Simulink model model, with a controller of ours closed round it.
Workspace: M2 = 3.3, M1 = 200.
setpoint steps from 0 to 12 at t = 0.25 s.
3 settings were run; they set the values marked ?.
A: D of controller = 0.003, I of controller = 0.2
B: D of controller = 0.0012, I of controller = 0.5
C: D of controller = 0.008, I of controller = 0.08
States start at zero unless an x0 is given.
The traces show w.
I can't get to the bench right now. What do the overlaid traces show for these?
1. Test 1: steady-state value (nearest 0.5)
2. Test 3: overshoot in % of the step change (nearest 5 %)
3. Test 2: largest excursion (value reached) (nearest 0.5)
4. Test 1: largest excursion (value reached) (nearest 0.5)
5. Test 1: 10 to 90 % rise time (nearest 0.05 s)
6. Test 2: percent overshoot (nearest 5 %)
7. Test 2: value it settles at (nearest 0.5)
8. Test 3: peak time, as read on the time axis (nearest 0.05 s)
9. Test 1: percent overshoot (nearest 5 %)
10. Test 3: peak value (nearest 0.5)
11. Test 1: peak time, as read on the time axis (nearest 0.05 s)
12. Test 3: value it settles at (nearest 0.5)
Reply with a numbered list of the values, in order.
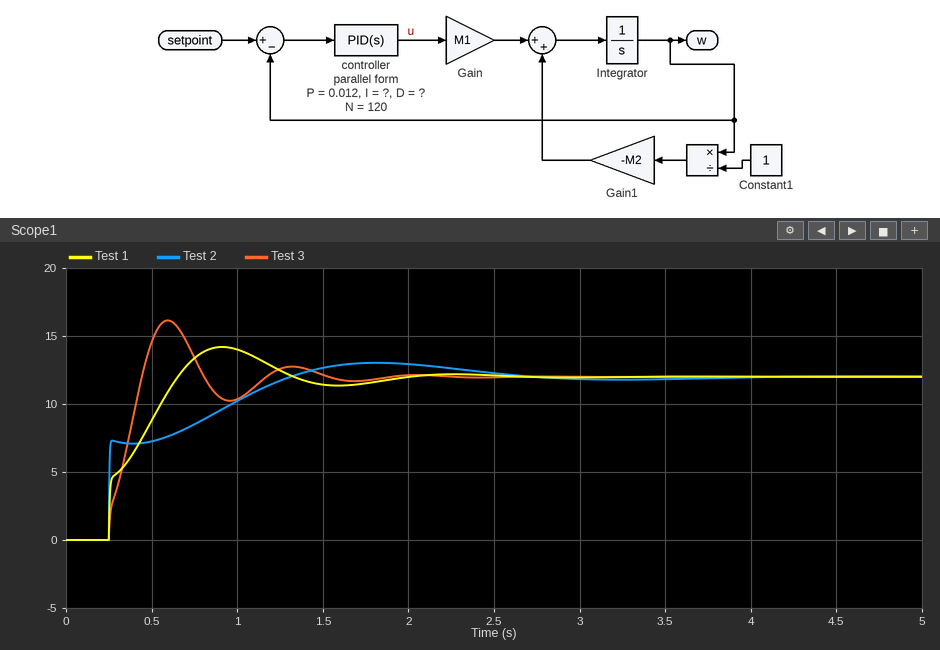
1. 12.0
2. 35 %
3. 13.0
4. 14.0
5. 0.35 s
6. 10 %
7. 12.0
8. 0.60 s
9. 20 %
10. 16.0
11. 0.90 s
12. 12.0
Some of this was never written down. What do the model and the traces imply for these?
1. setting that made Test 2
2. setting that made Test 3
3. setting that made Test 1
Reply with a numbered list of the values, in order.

1. C
2. B
3. A
